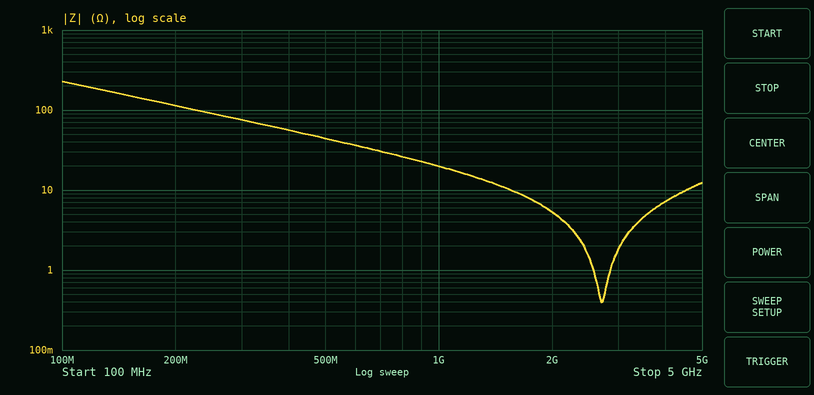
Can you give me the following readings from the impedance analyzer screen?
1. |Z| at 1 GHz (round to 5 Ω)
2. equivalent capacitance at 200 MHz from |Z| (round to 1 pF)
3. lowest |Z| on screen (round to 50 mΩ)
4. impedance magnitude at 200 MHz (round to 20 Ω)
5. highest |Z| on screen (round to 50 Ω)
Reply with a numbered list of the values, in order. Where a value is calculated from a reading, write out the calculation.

1. 20 Ω
2. C = 1/(2π × 200 MHz × 120 Ω) ≈ 7 pF
3. 400 mΩ
4. 120 Ω
5. 250 Ω
